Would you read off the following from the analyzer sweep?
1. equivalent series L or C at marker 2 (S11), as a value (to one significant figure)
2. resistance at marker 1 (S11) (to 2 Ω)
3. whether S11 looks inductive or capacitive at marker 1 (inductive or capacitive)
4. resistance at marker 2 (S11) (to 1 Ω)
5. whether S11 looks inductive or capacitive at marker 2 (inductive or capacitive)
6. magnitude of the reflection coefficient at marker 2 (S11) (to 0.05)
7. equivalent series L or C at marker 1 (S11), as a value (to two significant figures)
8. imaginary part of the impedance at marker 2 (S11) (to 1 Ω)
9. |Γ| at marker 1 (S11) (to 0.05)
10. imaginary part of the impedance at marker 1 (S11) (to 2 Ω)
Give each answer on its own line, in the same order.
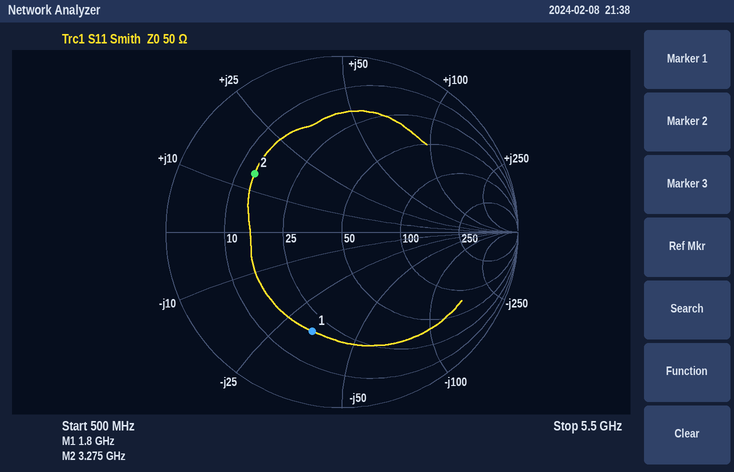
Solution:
700 pH
20 Ω
capacitive
14 Ω
inductive
0.60
2.6 pF
+14 Ω
0.60
-34 Ω
